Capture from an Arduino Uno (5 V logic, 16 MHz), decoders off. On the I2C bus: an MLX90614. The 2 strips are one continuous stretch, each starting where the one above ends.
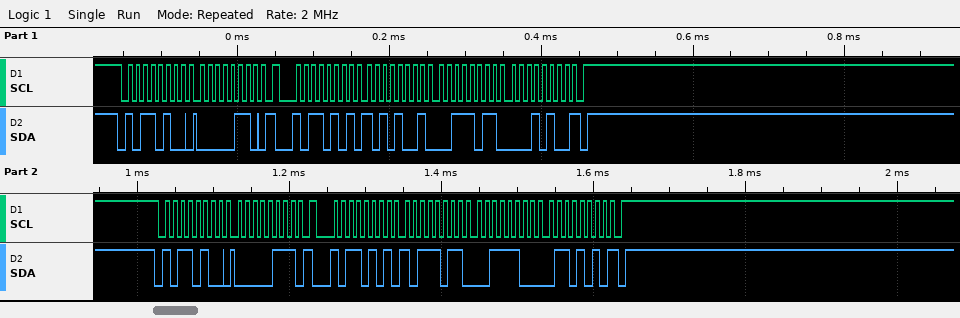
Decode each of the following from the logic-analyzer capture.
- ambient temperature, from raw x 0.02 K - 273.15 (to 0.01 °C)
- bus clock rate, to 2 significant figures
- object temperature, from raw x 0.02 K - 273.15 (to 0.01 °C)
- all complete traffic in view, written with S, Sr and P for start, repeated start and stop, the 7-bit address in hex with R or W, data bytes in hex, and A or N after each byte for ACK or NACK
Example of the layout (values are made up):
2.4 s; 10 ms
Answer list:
32.31 °C; 100 kHz; 37.79 °C; S 5AW A 06 A Sr 5AR A A9 A 3B A 14 N P S 5AW A 07 A Sr 5AR A BB A 3C A 6A N P
